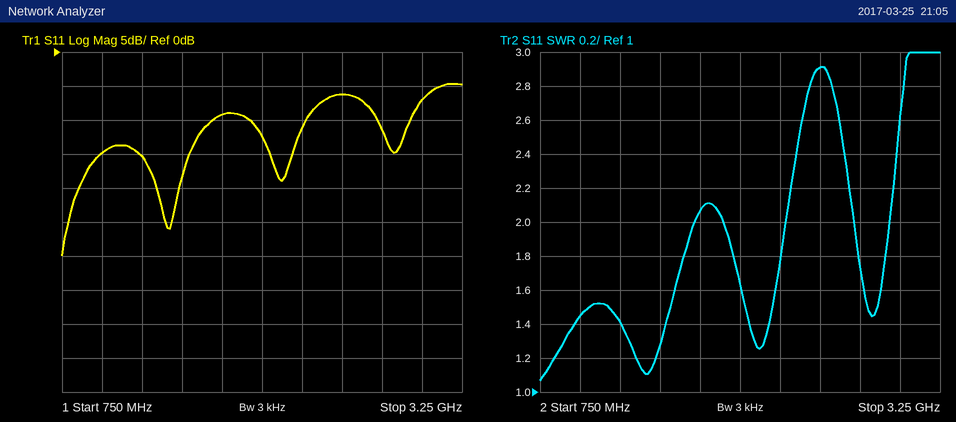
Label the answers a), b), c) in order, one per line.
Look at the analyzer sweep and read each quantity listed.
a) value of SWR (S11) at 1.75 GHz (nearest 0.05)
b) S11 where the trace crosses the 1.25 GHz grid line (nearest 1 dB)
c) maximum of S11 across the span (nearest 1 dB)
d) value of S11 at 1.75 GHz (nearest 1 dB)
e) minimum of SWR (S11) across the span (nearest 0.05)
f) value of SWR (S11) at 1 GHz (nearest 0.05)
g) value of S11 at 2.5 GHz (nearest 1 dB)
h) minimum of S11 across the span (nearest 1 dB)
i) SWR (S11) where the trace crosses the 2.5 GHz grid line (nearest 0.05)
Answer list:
a) 2.05
b) -15 dB
c) -5 dB
d) -9 dB
e) 1.05
f) 1.45
g) -6 dB
h) -30 dB
i) 2.90
